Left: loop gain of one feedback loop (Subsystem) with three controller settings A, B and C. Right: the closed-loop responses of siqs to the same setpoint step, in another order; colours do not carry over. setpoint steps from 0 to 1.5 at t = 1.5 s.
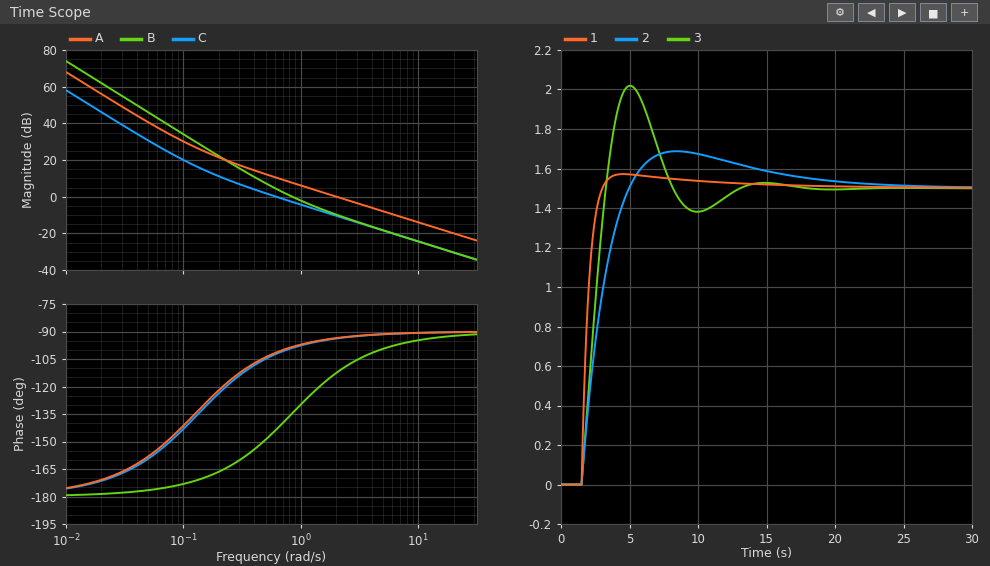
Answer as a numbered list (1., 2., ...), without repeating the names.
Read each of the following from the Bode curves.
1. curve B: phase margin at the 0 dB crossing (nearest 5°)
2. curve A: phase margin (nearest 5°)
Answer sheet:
1. 45°
2. 85°
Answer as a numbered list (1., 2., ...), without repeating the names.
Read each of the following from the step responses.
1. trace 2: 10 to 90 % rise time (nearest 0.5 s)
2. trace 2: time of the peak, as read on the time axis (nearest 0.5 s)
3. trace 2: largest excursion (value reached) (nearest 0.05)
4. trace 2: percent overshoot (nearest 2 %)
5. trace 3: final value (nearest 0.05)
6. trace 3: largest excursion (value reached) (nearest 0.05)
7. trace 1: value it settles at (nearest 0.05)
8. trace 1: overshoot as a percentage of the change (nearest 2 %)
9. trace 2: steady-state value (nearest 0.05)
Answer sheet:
1. 2.5 s
2. 8.5 s
3. 1.70
4. 12 %
5. 1.50
6. 2.00
7. 1.50
8. 4 %
9. 1.50
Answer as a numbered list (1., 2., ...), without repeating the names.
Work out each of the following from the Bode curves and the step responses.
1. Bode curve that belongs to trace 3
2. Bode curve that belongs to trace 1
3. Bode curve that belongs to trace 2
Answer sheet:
1. B
2. A
3. C
